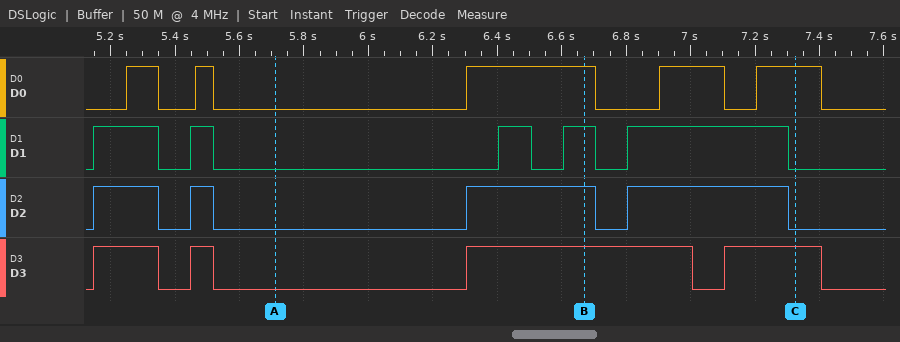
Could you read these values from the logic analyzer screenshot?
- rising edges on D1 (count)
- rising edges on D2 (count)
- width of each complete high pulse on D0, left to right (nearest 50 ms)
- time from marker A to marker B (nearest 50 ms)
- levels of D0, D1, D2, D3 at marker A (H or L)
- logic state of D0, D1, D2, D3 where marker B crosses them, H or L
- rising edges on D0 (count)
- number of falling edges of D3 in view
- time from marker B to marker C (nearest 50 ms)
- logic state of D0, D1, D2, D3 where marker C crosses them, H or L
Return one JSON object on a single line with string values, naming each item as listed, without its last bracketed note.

{"rising edges on D1": "5", "rising edges on D2": "4", "width of each complete high pulse on D0, left to right": "100 ms, 50 ms, 400 ms, 200 ms, 200 ms", "time from marker A to marker B": "950 ms", "levels of D0, D1, D2, D3 at marker A": "D0=L, D1=L, D2=L, D3=L", "logic state of D0, D1, D2, D3 where marker B crosses them, H or L": "D0=H, D1=H, D2=H, D3=H", "rising edges on D0": "5", "number of falling edges of D3 in view": "4", "time from marker B to marker C": "650 ms", "logic state of D0, D1, D2, D3 where marker C crosses them, H or L": "D0=H, D1=L, D2=L, D3=H"}
